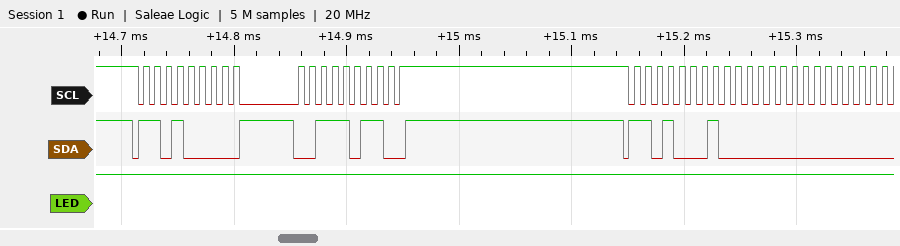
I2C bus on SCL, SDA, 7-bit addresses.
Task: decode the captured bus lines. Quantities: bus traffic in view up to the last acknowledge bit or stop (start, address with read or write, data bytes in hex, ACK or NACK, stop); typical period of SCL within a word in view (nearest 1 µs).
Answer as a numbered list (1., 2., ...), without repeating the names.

1. start, address 68 write ACK, 3B ACK, stop, start, address 68 read ACK, 00 ACK
2. 10 µs
